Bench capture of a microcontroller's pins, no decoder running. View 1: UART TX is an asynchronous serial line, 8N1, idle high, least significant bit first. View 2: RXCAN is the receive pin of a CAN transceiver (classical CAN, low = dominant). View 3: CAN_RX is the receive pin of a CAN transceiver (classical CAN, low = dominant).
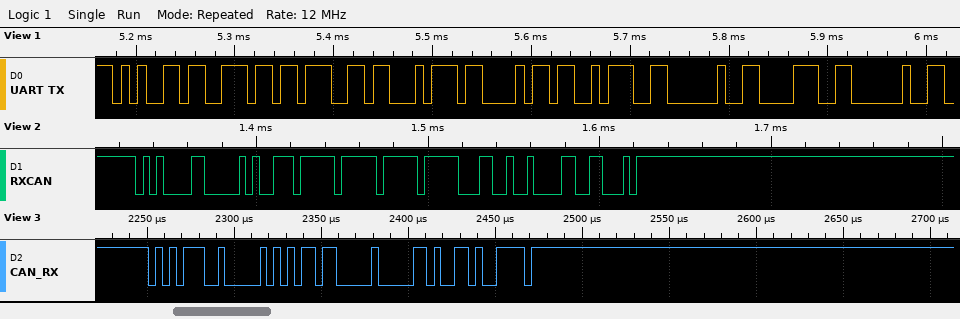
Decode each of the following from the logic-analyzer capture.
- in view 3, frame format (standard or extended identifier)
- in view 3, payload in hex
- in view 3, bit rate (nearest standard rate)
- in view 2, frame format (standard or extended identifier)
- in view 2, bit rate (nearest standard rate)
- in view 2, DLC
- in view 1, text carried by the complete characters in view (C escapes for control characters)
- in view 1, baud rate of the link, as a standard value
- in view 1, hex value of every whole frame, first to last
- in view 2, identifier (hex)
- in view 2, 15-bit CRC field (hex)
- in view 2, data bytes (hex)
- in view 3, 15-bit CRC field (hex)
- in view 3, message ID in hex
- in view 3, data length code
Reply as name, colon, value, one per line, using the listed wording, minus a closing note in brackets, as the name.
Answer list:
in view 3, frame format: standard
in view 3, payload in hex: B6 00
in view 3, bit rate: 250 kbit/s
in view 2, frame format: standard
in view 2, bit rate: 250 kbit/s
in view 2, DLC: 4
in view 1, text carried by the complete characters in view: "ength: 8 "
in view 1, baud rate of the link, as a standard value: 115200 baud
in view 1, hex value of every whole frame, first to last: 65 6E 67 74 68 3A 20 38 20
in view 2, identifier: 0x50C
in view 2, 15-bit CRC field: 0x2198
in view 2, data bytes: EF FF FF 32
in view 3, 15-bit CRC field: 0x29A7
in view 3, message ID in hex: 0x572
in view 3, data length code: 2
